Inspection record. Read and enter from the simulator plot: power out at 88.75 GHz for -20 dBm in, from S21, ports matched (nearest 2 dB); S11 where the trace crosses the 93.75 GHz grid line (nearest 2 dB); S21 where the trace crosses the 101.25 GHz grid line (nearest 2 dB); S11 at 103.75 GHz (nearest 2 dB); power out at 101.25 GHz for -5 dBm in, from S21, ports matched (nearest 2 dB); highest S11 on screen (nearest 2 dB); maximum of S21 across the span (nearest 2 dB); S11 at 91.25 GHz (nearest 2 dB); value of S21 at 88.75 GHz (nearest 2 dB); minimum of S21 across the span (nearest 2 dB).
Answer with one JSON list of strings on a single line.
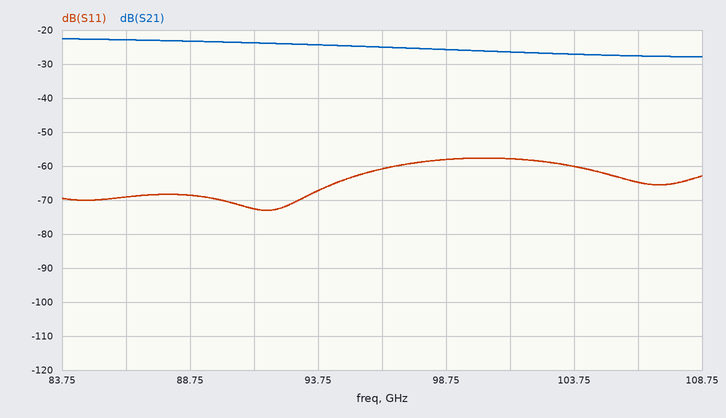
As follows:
["-44 dBm", "-68 dB", "-26 dB", "-60 dB", "-32 dBm", "-58 dB", "-22 dB", "-72 dB", "-24 dB", "-28 dB"]
